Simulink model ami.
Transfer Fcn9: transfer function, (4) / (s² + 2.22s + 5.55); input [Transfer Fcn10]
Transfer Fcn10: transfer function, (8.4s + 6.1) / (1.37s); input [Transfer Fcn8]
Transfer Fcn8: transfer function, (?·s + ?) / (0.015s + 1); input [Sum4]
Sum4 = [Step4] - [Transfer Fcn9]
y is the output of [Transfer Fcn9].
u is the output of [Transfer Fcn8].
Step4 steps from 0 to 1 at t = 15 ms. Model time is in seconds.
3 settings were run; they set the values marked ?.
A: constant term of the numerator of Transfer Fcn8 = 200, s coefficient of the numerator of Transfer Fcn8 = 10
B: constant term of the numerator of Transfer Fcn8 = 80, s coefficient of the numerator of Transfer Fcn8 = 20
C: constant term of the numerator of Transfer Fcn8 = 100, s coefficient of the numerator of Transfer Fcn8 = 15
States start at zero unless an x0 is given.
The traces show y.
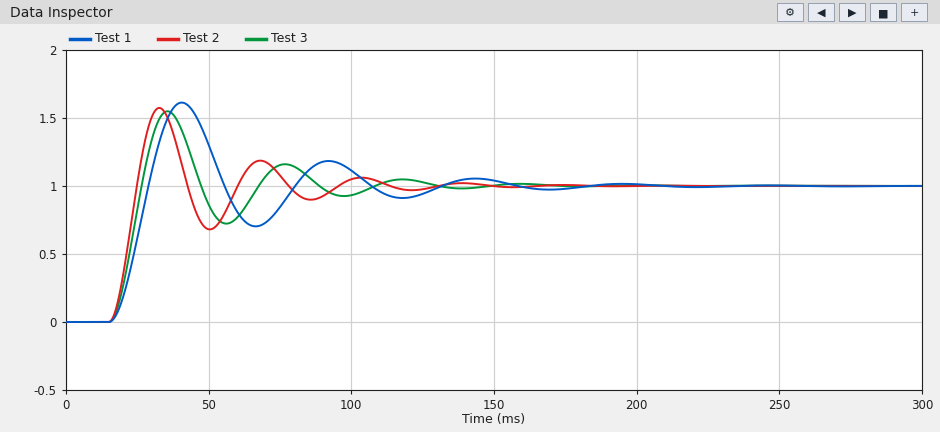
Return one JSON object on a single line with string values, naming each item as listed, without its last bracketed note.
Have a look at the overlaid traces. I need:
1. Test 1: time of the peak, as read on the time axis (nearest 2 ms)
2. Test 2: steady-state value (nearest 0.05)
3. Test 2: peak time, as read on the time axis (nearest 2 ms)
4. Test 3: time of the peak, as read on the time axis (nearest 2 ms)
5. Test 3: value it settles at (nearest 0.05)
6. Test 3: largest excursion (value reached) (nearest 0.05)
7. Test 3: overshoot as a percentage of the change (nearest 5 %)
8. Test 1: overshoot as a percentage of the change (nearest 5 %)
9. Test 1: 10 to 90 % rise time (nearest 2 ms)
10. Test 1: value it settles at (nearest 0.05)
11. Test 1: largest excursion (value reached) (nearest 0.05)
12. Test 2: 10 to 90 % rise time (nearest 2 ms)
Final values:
{"Test 1: time of the peak, as read on the time axis": "40 ms", "Test 2: steady-state value": "1.00", "Test 2: peak time, as read on the time axis": "32 ms", "Test 3: time of the peak, as read on the time axis": "36 ms", "Test 3: value it settles at": "1.00", "Test 3: largest excursion (value reached)": "1.55", "Test 3: overshoot as a percentage of the change": "55 %", "Test 1: overshoot as a percentage of the change": "60 %", "Test 1: 10 to 90 % rise time": "10 ms", "Test 1: value it settles at": "1.00", "Test 1: largest excursion (value reached)": "1.60", "Test 2: 10 to 90 % rise time": "6 ms"}
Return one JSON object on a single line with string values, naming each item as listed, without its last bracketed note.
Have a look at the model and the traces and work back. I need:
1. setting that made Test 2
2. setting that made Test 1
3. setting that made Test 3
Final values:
{"setting that made Test 2": "B", "setting that made Test 1": "A", "setting that made Test 3": "C"}
